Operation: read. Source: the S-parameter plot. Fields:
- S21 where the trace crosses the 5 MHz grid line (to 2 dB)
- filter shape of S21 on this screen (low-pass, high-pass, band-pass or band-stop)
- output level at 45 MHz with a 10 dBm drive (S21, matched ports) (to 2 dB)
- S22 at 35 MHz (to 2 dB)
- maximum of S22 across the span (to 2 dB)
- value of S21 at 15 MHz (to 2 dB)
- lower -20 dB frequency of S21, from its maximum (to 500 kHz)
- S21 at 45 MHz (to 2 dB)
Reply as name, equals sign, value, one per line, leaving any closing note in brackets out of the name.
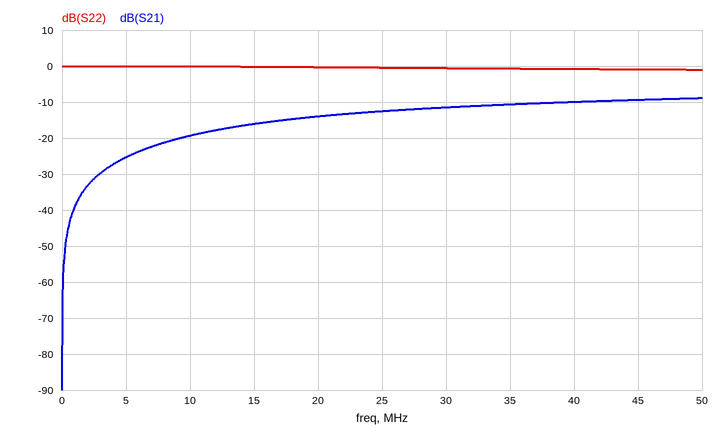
S21 where the trace crosses the 5 MHz grid line = -26 dB
filter shape of S21 on this screen = high-pass
output level at 45 MHz with a 10 dBm drive (S21, matched ports) = 0 dBm
S22 at 35 MHz = 0 dB
maximum of S22 across the span = 0 dB
value of S21 at 15 MHz = -16 dB
lower -20 dB frequency of S21, from its maximum = 3.5 MHz
S21 at 45 MHz = -10 dB
